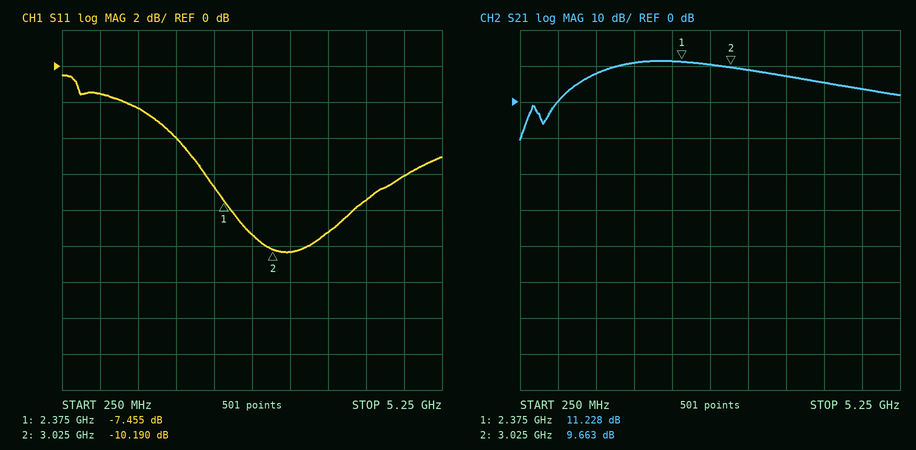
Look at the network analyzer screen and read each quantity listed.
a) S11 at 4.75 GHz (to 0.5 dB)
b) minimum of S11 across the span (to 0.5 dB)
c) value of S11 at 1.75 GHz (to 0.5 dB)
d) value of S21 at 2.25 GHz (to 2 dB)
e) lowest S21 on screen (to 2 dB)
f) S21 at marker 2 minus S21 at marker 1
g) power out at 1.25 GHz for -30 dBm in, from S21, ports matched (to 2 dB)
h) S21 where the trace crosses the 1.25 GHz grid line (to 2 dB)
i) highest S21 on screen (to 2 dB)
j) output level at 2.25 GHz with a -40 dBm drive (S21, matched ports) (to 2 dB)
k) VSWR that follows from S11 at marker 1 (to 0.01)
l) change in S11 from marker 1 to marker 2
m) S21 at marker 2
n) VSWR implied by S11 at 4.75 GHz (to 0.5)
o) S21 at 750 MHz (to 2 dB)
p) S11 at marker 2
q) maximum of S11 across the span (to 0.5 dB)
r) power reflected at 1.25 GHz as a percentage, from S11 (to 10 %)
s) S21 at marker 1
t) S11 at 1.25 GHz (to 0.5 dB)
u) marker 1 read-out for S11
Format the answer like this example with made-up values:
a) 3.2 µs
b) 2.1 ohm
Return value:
a) -6.0 dB
b) -10.5 dB
c) -4.0 dB
d) 12 dB
e) -10 dB
f) -1.565 dB
g) -22 dBm
h) 8 dB
i) 12 dB
j) -28 dBm
k) 2.47
l) -2.735 dB
m) 9.663 dB
n) 3.0
o) 0 dB
p) -10.190 dB
q) -0.5 dB
r) 60 %
s) 11.228 dB
t) -2.5 dB
u) -7.455 dB
